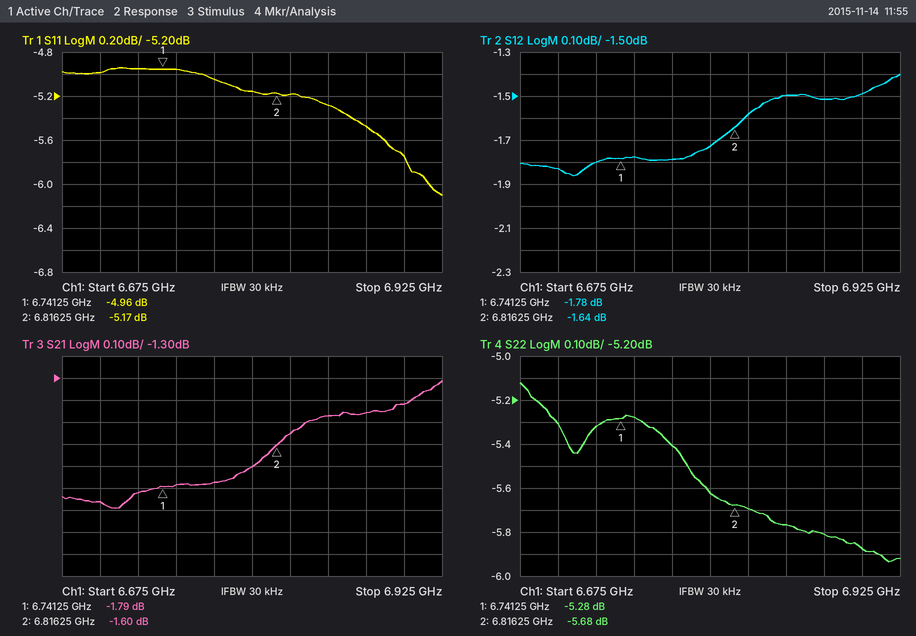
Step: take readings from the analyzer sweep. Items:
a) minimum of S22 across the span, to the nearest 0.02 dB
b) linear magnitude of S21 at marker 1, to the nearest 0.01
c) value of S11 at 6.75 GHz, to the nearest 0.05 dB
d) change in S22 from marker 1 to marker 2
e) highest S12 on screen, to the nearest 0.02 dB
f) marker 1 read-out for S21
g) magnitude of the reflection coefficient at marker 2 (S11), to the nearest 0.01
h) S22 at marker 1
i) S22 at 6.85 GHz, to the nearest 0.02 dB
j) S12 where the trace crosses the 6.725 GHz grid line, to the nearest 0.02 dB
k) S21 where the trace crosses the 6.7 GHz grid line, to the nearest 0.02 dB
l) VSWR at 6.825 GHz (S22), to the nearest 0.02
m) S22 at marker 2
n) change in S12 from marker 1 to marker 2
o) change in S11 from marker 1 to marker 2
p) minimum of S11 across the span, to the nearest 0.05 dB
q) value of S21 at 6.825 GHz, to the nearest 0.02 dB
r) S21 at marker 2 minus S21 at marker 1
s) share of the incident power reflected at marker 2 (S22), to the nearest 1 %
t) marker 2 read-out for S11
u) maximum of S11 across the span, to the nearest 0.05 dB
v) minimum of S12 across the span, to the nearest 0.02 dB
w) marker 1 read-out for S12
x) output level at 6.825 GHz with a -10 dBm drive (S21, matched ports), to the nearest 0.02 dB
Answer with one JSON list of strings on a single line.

["-5.94 dB", "0.81", "-4.95 dB", "-0.40 dB", "-1.40 dB", "-1.79 dB", "0.55", "-5.28 dB", "-5.76 dB", "-1.80 dB", "-1.86 dB", "3.16", "-5.68 dB", "0.14 dB", "-0.21 dB", "-6.10 dB", "-1.56 dB", "0.19 dB", "27 %", "-5.17 dB", "-4.95 dB", "-1.86 dB", "-1.78 dB", "-11.56 dBm"]
